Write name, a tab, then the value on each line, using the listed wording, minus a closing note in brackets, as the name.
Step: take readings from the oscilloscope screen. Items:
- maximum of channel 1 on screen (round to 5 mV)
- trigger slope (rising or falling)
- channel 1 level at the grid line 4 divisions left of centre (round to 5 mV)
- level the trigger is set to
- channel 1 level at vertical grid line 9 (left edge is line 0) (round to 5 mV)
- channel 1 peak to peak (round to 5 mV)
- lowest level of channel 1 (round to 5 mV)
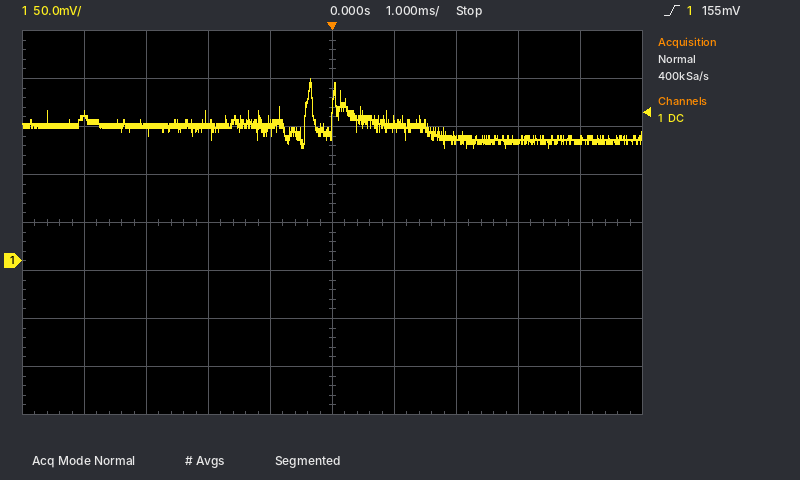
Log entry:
maximum of channel 1 on screen	190 mV
trigger slope	rising
channel 1 level at the grid line 4 divisions left of centre	150 mV
level the trigger is set to	155 mV
channel 1 level at vertical grid line 9 (left edge is line 0)	125 mV
channel 1 peak to peak	70 mV
lowest level of channel 1	120 mV
